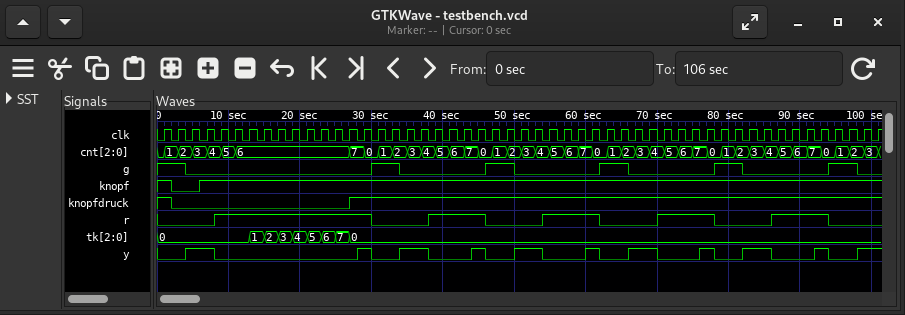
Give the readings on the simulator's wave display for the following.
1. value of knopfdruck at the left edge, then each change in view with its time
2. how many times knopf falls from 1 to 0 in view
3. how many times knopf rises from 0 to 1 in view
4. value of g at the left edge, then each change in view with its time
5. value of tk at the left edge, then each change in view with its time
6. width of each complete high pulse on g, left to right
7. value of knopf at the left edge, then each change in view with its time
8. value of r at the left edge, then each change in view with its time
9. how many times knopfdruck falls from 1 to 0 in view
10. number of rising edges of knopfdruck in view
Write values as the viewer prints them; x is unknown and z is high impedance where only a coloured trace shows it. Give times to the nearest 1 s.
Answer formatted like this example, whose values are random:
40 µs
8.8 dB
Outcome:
1, 0 at 2 s, 1 at 27 s
1
1
1, 0 at 4 s, 1 at 30 s, 0 at 34 s, 1 at 46 s, 0 at 50 s, 1 at 62 s, 0 at 66 s, 1 at 78 s, 0 at 82 s, 1 at 94 s, 0 at 98 s
0, 1 at 13 s, 2 at 15 s, 3 at 17 s, 4 at 19 s, 5 at 21 s, 6 at 23 s, 7 at 25 s, 0 at 27 s
4 s, 4 s, 4 s, 4 s, 4 s
1, 0 at 2 s, 1 at 6 s
0, 1 at 8 s, 0 at 30 s, 1 at 38 s, 0 at 46 s, 1 at 54 s, 0 at 62 s, 1 at 70 s, 0 at 78 s, 1 at 86 s, 0 at 94 s
1
1
